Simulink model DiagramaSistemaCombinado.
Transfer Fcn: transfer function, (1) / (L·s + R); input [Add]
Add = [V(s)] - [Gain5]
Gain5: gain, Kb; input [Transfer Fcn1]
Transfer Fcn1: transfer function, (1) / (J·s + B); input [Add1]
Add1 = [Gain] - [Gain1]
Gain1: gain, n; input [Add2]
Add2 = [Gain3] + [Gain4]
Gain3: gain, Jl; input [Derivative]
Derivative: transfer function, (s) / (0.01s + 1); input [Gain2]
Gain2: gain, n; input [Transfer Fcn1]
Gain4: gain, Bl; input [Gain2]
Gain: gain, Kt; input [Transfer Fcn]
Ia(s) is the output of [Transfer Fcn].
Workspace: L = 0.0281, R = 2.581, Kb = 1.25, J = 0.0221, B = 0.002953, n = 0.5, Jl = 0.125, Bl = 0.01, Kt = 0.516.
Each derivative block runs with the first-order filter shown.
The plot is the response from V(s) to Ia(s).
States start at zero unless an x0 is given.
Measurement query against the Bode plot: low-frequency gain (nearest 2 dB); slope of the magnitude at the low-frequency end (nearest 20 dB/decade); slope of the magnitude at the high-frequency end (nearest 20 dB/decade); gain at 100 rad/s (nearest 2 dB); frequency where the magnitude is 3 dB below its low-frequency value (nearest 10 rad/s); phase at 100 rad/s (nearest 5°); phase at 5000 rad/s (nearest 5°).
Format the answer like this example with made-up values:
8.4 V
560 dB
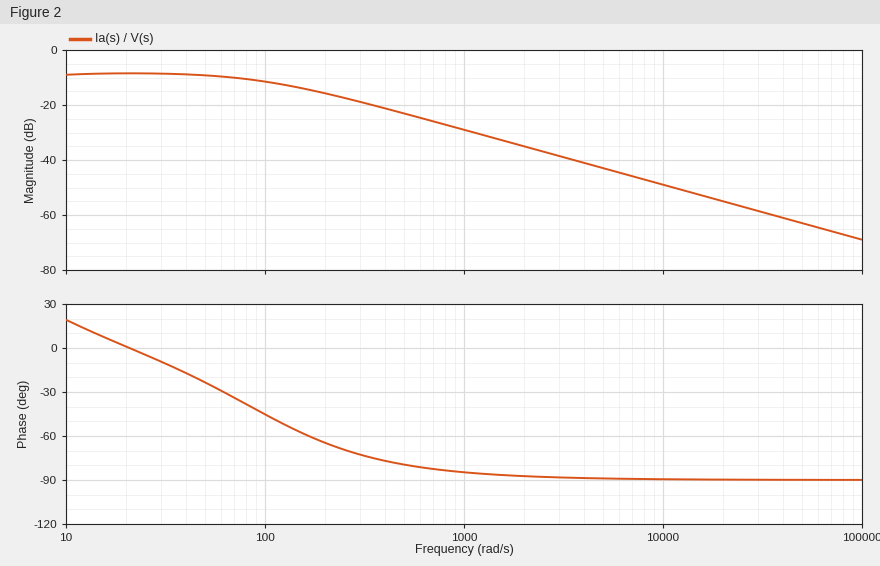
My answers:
-8 dB
0 dB/decade
-20 dB/decade
-12 dB
100 rad/s
-45°
-90°
